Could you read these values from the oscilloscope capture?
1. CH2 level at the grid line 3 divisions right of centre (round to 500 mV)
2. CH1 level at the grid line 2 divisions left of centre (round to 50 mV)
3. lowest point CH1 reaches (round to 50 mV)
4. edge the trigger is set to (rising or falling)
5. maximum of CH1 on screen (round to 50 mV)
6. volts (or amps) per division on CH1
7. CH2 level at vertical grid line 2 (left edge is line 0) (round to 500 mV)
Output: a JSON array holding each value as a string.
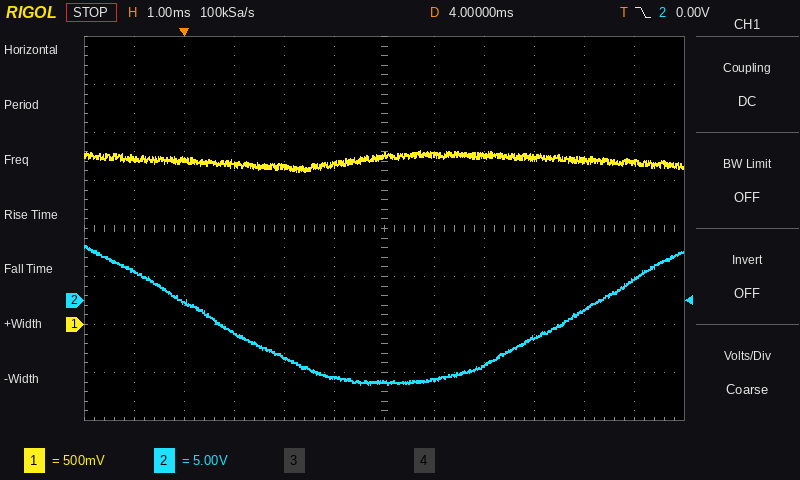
["-4.0 V", "1.65 V", "1.60 V", "falling", "1.80 V", "500 mV", "0.0 V"]
